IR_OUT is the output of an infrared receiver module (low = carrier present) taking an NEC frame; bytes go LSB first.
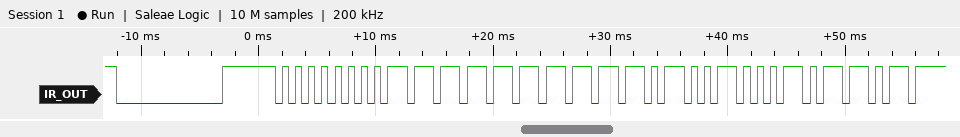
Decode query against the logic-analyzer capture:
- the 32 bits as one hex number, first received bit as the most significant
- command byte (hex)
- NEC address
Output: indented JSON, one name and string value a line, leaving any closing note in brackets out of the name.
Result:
{
  "the 32 bits as one hex number, first received bit as the most significant": "0x00FFD22D",
  "command byte": "0x4B",
  "NEC address": "0x00"
}
